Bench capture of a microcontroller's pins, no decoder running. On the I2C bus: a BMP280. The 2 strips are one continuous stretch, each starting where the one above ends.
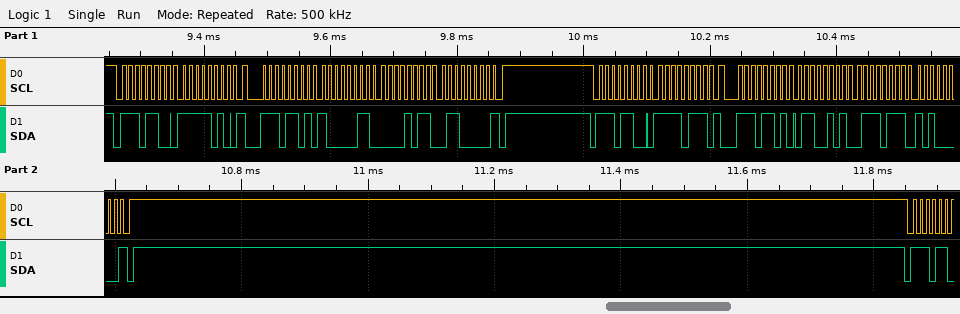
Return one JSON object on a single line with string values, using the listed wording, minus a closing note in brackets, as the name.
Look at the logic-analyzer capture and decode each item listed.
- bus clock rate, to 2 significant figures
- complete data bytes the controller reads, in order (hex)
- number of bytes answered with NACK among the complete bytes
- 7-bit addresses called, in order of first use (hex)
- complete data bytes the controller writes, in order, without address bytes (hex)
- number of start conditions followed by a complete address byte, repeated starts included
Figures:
{"bus clock rate, to 2 significant figures": "100 kHz", "complete data bytes the controller reads, in order": "83 0B 60 65 77 A0", "number of bytes answered with NACK among the complete bytes": "2", "7-bit addresses called, in order of first use": "0x76", "complete data bytes the controller writes, in order, without address bytes": "FA F7", "number of start conditions followed by a complete address byte, repeated starts included": "4"}
